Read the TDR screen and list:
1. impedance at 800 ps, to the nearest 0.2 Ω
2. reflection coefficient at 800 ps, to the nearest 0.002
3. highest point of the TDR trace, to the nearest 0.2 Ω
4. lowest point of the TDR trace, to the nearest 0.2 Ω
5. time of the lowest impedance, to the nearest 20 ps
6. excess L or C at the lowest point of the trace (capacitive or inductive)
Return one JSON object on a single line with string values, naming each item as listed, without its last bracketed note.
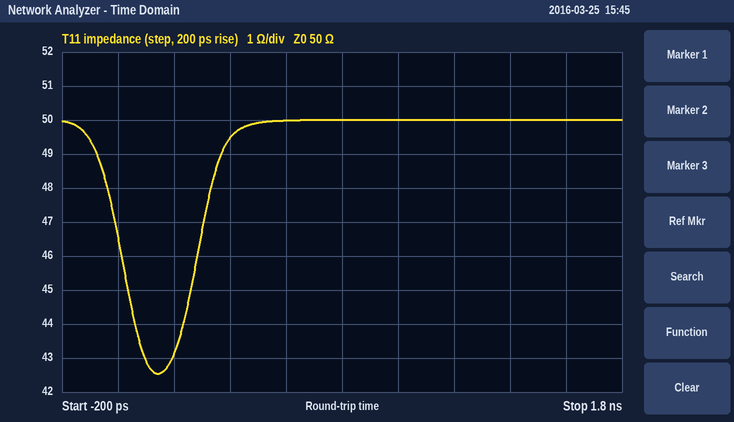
{"impedance at 800 ps, to the nearest 0.2 Ω": "50.0 Ω", "reflection coefficient at 800 ps, to the nearest 0.002": "0.000", "highest point of the TDR trace, to the nearest 0.2 Ω": "50.0 Ω", "lowest point of the TDR trace, to the nearest 0.2 Ω": "42.6 Ω", "time of the lowest impedance, to the nearest 20 ps": "140 ps", "excess L or C at the lowest point of the trace": "capacitive"}
